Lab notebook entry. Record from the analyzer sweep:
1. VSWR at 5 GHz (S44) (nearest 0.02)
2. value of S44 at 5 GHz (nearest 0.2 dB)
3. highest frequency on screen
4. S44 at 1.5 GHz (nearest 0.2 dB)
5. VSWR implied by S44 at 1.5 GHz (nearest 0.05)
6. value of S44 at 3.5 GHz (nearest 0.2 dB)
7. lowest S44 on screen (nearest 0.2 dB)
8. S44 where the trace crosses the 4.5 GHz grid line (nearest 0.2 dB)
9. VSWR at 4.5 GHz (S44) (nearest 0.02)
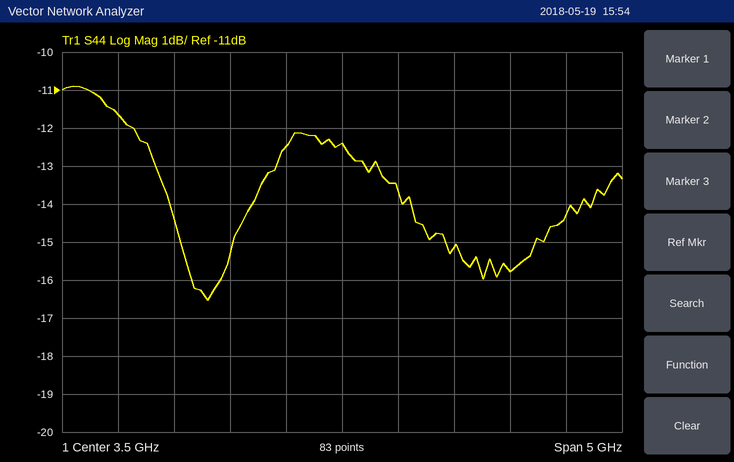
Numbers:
1.38
-15.8 dB
6 GHz
-11.6 dB
1.70
-12.4 dB
-16.6 dB
-15.2 dB
1.42
